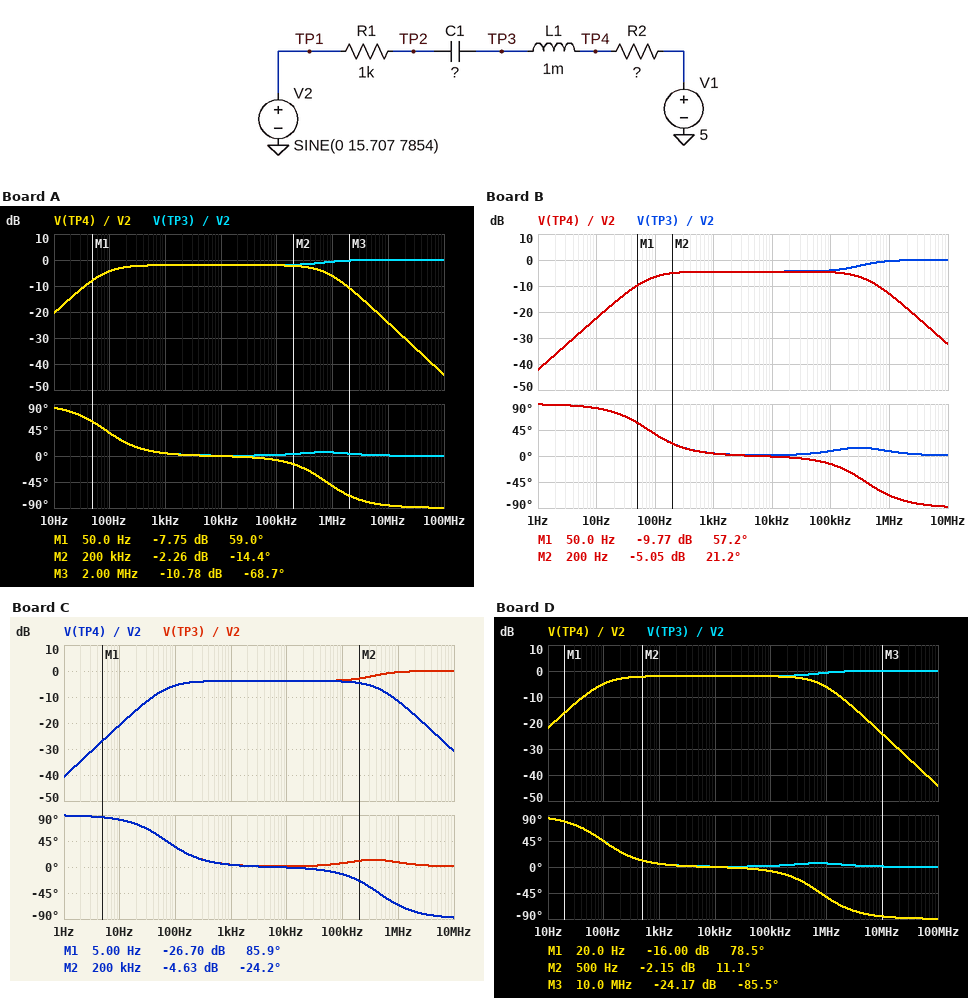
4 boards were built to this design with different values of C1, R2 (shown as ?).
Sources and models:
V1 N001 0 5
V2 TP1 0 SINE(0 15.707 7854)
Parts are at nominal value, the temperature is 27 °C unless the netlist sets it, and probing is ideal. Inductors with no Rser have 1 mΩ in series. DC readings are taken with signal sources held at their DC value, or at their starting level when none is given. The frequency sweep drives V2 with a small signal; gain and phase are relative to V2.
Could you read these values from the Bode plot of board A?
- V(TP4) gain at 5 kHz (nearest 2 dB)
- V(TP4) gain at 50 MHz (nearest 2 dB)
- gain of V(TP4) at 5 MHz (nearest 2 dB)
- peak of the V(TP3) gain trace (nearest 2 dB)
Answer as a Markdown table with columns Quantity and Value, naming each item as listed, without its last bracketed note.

| Quantity | Value |
|---|---|
| V(TP4) gain at 5 kHz | -2 dB |
| V(TP4) gain at 50 MHz | -38 dB |
| gain of V(TP4) at 5 MHz | -18 dB |
| peak of the V(TP3) gain trace | 0 dB |
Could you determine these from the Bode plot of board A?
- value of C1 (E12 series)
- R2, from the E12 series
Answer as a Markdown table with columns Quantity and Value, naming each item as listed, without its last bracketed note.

| Quantity | Value |
|---|---|
| value of C1 | 390 nF |
| R2, from the E12 series | 3.9 kΩ |
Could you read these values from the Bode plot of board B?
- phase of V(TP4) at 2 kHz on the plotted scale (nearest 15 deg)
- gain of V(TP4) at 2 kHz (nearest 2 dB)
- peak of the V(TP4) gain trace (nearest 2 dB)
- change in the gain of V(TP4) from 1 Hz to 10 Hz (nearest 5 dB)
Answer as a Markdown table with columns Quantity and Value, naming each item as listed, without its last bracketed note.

| Quantity | Value |
|---|---|
| phase of V(TP4) at 2 kHz on the plotted scale | 0 deg |
| gain of V(TP4) at 2 kHz | -4 dB |
| peak of the V(TP4) gain trace | -4 dB |
| change in the gain of V(TP4) from 1 Hz to 10 Hz | 20 dB |
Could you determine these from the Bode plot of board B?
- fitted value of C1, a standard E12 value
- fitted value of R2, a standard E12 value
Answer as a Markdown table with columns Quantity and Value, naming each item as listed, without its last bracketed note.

| Quantity | Value |
|---|---|
| fitted value of C1, a standard E12 value | 820 nF |
| fitted value of R2, a standard E12 value | 1.5 kΩ |
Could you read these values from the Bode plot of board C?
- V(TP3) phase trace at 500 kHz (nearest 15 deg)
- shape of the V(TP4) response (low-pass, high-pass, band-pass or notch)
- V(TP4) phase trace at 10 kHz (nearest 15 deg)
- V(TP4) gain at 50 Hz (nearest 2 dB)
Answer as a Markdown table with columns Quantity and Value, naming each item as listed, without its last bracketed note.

| Quantity | Value |
|---|---|
| V(TP3) phase trace at 500 kHz | 15 deg |
| shape of the V(TP4) response | band-pass |
| V(TP4) phase trace at 10 kHz | 0 deg |
| V(TP4) gain at 50 Hz | -8 dB |
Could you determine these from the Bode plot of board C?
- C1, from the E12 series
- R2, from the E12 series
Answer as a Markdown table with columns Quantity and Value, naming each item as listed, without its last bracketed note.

| Quantity | Value |
|---|---|
| C1, from the E12 series | 820 nF |
| R2, from the E12 series | 1.8 kΩ |
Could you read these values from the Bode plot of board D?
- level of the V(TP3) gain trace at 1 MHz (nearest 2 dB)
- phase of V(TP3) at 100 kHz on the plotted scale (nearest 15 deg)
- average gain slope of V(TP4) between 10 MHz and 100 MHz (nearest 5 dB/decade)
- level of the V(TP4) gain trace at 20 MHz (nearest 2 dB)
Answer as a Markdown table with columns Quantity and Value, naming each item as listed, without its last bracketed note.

| Quantity | Value |
|---|---|
| level of the V(TP3) gain trace at 1 MHz | 0 dB |
| phase of V(TP3) at 100 kHz on the plotted scale | 0 deg |
| average gain slope of V(TP4) between 10 MHz and 100 MHz | -20 dB/decade |
| level of the V(TP4) gain trace at 20 MHz | -30 dB |
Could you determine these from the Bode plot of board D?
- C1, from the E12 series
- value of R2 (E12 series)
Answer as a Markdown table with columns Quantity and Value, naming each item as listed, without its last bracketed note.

| Quantity | Value |
|---|---|
| C1, from the E12 series | 330 nF |
| value of R2 | 3.9 kΩ |
